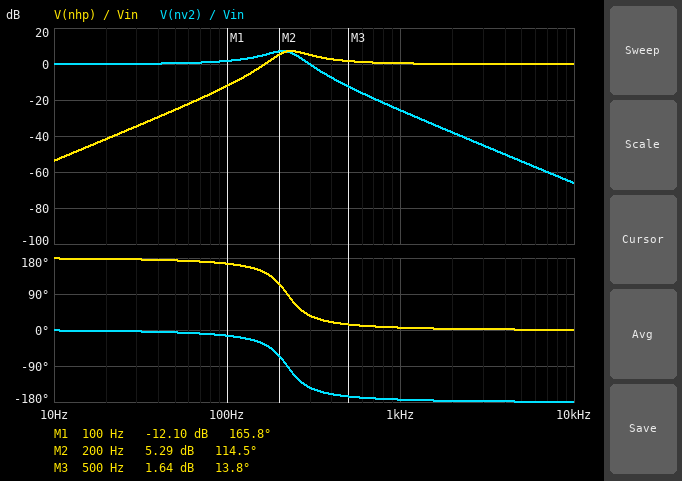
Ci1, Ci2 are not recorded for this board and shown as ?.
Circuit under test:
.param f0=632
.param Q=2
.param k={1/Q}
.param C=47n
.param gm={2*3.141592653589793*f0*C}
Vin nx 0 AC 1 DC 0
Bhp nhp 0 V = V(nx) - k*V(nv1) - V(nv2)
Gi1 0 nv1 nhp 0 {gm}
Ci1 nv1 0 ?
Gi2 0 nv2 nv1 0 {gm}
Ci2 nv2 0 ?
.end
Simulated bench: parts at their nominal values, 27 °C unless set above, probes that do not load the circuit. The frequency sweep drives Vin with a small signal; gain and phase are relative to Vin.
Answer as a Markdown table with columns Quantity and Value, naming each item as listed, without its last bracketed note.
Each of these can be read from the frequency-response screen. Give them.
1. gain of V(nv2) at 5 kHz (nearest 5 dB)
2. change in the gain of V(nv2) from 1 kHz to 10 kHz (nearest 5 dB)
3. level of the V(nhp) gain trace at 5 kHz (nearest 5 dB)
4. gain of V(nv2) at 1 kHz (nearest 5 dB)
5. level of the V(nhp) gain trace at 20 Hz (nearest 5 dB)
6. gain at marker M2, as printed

| Quantity | Value |
|---|---|
| gain of V(nv2) at 5 kHz | -55 dB |
| change in the gain of V(nv2) from 1 kHz to 10 kHz | -40 dB |
| level of the V(nhp) gain trace at 5 kHz | 0 dB |
| gain of V(nv2) at 1 kHz | -25 dB |
| level of the V(nhp) gain trace at 20 Hz | -40 dB |
| gain at marker M2, as printed | 5.29 dB |
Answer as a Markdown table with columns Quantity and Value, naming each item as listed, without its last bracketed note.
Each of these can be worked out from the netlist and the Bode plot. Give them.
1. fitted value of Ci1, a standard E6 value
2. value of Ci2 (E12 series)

| Quantity | Value |
|---|---|
| fitted value of Ci1, a standard E6 value | 150 nF |
| value of Ci2 | 120 nF |
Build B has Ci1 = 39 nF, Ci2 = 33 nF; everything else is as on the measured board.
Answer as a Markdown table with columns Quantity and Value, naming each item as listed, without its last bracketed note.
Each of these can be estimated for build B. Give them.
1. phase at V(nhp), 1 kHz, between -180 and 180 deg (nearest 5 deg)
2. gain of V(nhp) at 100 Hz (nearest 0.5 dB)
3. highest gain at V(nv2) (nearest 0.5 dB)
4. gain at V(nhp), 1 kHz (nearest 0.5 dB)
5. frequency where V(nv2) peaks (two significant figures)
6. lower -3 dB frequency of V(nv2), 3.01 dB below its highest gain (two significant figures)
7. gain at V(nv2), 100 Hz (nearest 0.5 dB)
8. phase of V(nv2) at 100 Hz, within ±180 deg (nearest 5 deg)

| Quantity | Value |
|---|---|
| phase at V(nhp), 1 kHz, between -180 and 180 deg | 50 deg |
| gain of V(nhp) at 100 Hz | -36.5 dB |
| highest gain at V(nv2) | 7.0 dB |
| gain at V(nhp), 1 kHz | 6.0 dB |
| frequency where V(nv2) peaks | 780 Hz |
| lower -3 dB frequency of V(nv2), 3.01 dB below its highest gain | 550 Hz |
| gain at V(nv2), 100 Hz | 0 dB |
| phase of V(nv2) at 100 Hz, within ±180 deg | -5 deg |
